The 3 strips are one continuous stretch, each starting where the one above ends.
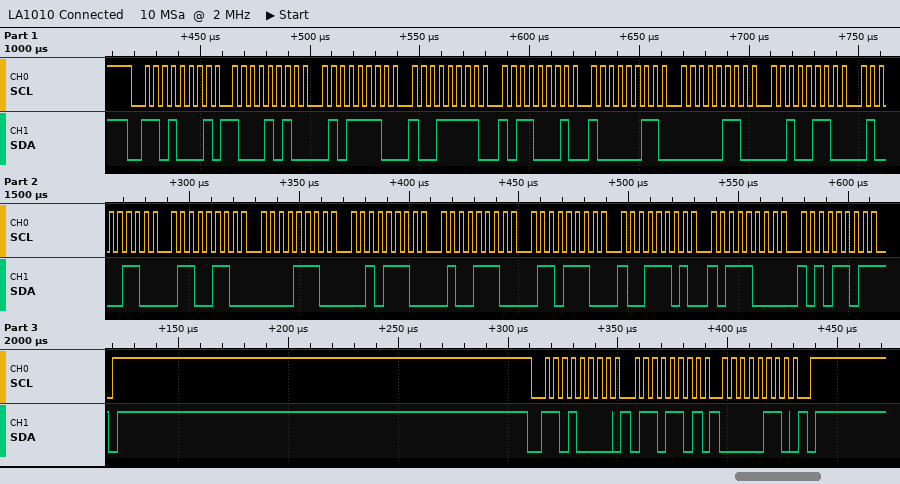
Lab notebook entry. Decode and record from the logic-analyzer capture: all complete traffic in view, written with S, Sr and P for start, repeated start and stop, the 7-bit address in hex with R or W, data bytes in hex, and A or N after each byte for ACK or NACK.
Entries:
S 68R A 8A A 5E A 9F A B1 A 83 A 06 A 26 A 46 A 66 A 0E A 2E A 4E A 6E A 9D A B8 A AD N P S 68W A 6D A 06 A P
